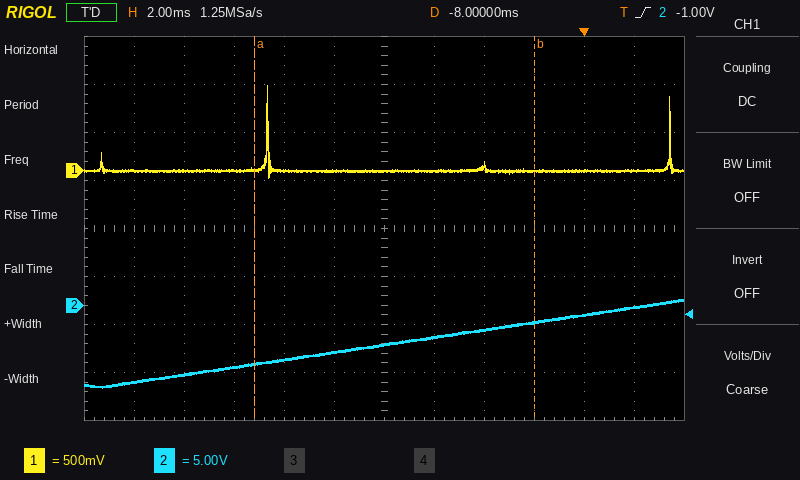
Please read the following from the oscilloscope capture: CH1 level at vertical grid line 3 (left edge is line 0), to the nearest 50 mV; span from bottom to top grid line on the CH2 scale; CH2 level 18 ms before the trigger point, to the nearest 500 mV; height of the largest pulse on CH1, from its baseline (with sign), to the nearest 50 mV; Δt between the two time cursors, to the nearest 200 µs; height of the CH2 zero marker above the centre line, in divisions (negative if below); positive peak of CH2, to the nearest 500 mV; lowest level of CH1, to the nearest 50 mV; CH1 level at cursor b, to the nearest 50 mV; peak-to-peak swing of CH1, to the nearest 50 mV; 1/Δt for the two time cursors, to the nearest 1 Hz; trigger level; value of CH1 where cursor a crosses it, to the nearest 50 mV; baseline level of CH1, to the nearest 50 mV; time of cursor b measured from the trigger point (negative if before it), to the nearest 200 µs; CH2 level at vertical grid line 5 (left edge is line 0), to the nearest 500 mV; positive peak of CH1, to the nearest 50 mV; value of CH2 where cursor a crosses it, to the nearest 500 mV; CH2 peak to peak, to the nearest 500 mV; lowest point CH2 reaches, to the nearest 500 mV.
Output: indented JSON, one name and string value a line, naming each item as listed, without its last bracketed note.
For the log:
{
  "CH1 level at vertical grid line 3 (left edge is line 0), to the nearest 50 mV": "0 mV",
  "span from bottom to top grid line on the CH2 scale": "40 V",
  "CH2 level 18 ms before the trigger point, to the nearest 500 mV": "-8.0 V",
  "height of the largest pulse on CH1, from its baseline (with sign), to the nearest 50 mV": "+900 mV",
  "Δt between the two time cursors, to the nearest 200 µs": "11.2 ms",
  "height of the CH2 zero marker above the centre line, in divisions": "-1.6 div",
  "positive peak of CH2, to the nearest 500 mV": "500 mV",
  "lowest level of CH1, to the nearest 50 mV": "-50 mV",
  "CH1 level at cursor b, to the nearest 50 mV": "0 mV",
  "peak-to-peak swing of CH1, to the nearest 50 mV": "950 mV",
  "1/Δt for the two time cursors, to the nearest 1 Hz": "89 Hz",
  "trigger level": "-1.00 V",
  "value of CH1 where cursor a crosses it, to the nearest 50 mV": "0 mV",
  "baseline level of CH1, to the nearest 50 mV": "0 mV",
  "time of cursor b measured from the trigger point (negative if before it), to the nearest 200 µs": "-2.0 ms",
  "CH2 level at vertical grid line 5 (left edge is line 0), to the nearest 500 mV": "-5.0 V",
  "positive peak of CH1, to the nearest 50 mV": "900 mV",
  "value of CH2 where cursor a crosses it, to the nearest 500 mV": "-6.0 V",
  "CH2 peak to peak, to the nearest 500 mV": "9.0 V",
  "lowest point CH2 reaches, to the nearest 500 mV": "-8.5 V"
}
